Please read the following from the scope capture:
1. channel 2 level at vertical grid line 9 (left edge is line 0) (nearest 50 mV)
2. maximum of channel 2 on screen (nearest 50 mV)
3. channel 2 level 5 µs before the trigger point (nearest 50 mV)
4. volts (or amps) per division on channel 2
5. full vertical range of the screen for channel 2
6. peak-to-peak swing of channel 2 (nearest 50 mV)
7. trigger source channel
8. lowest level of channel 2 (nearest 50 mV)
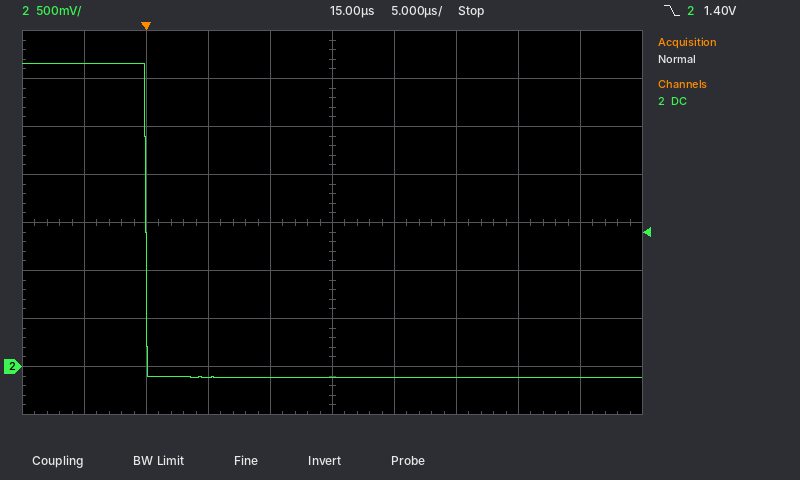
-100 mV
3.15 V
3.15 V
500 mV
4 V
3.25 V
channel 2
-100 mV
